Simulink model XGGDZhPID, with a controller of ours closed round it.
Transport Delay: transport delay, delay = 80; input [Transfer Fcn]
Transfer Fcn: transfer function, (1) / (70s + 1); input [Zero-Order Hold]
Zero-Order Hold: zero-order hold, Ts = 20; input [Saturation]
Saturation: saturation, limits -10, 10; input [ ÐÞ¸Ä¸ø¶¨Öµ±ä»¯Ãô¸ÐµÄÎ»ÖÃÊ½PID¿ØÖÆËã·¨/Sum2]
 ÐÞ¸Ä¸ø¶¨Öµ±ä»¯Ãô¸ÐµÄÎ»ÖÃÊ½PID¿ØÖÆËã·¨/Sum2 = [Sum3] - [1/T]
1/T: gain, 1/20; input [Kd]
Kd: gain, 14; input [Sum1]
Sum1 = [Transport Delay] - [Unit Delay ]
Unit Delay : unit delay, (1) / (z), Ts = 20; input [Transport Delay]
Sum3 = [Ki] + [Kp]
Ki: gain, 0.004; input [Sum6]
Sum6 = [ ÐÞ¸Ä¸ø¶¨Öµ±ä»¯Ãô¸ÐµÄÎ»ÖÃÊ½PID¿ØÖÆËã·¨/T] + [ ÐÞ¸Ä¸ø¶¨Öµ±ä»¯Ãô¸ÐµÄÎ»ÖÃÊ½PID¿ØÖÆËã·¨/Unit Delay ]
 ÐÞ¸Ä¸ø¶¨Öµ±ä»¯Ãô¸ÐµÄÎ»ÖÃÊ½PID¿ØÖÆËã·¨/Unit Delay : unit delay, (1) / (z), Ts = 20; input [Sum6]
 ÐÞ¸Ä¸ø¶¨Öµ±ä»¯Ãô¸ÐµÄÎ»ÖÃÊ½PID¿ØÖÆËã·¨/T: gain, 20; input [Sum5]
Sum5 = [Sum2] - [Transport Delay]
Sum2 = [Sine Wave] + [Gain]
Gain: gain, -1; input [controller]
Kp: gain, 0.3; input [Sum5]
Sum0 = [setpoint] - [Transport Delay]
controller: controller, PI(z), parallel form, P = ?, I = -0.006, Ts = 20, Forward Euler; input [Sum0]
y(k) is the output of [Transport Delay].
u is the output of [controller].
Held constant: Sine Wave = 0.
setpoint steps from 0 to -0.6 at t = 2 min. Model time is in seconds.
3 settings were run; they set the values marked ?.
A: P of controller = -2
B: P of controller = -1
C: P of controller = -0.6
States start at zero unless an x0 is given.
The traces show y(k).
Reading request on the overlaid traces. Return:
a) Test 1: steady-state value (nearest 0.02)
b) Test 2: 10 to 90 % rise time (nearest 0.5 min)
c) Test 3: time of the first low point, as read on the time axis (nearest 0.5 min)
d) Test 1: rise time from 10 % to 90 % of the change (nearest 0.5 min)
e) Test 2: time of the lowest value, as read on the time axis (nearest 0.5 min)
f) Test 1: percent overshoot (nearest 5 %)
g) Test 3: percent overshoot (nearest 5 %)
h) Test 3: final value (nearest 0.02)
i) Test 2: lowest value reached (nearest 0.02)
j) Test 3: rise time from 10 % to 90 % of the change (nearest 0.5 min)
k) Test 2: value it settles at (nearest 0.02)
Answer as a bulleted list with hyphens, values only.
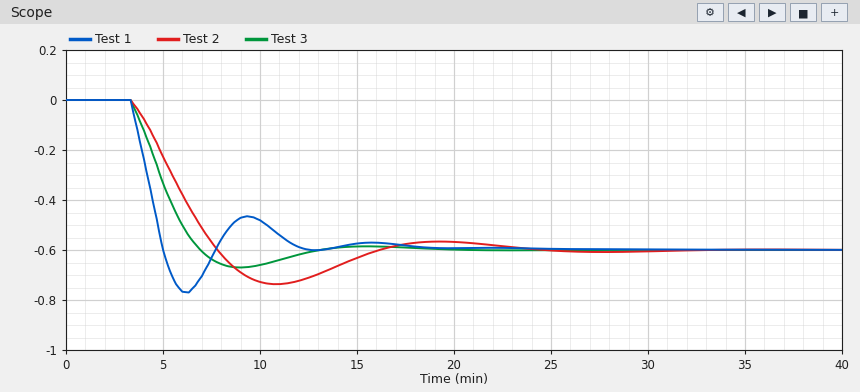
- -0.60
- 3.5 min
- 9.0 min
- 1.5 min
- 11.0 min
- 30 %
- 10 %
- -0.60
- -0.74
- 2.5 min
- -0.60
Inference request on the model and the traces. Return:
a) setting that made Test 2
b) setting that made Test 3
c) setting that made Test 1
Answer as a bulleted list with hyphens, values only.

- C
- B
- A
